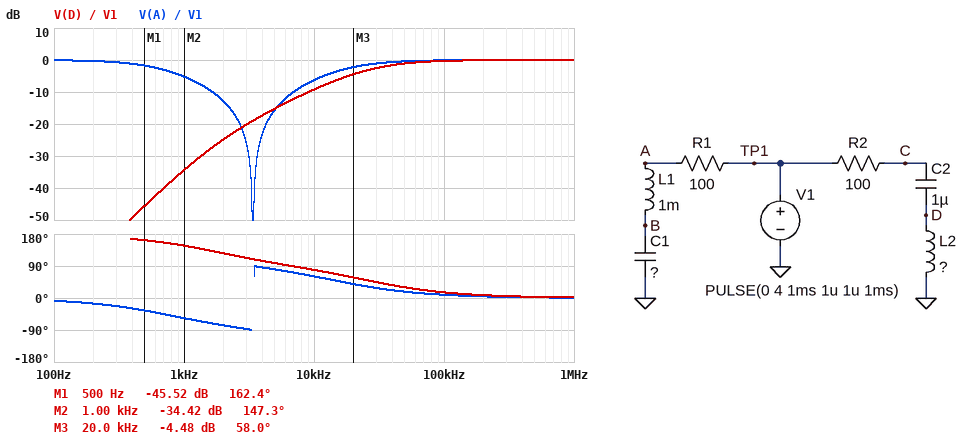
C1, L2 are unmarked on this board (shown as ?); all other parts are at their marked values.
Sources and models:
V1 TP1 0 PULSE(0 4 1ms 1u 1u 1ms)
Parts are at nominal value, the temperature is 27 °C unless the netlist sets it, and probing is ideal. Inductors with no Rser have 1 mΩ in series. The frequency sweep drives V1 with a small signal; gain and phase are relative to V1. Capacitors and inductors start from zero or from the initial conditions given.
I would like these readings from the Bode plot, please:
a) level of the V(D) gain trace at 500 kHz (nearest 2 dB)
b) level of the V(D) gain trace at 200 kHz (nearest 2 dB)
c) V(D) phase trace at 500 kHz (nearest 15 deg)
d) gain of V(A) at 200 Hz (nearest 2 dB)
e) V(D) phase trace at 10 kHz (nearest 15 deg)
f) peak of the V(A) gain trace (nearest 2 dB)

0 dB
0 dB
0 deg
0 dB
75 deg
0 dB
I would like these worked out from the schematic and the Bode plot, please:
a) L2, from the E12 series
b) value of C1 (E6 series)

560 µH
2.2 µF
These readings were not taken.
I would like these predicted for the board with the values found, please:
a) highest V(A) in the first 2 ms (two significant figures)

4.0 V
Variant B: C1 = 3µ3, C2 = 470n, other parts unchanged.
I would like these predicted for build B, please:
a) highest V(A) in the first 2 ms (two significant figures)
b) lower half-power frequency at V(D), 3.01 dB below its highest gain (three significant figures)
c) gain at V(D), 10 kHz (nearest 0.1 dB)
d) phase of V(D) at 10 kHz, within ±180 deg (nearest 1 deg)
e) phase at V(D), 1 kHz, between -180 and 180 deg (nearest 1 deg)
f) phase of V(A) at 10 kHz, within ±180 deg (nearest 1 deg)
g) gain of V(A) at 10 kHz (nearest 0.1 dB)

3.8 V
25.1 kHz
-9.1 dB
89 deg
163 deg
60 deg
-6.0 dB
